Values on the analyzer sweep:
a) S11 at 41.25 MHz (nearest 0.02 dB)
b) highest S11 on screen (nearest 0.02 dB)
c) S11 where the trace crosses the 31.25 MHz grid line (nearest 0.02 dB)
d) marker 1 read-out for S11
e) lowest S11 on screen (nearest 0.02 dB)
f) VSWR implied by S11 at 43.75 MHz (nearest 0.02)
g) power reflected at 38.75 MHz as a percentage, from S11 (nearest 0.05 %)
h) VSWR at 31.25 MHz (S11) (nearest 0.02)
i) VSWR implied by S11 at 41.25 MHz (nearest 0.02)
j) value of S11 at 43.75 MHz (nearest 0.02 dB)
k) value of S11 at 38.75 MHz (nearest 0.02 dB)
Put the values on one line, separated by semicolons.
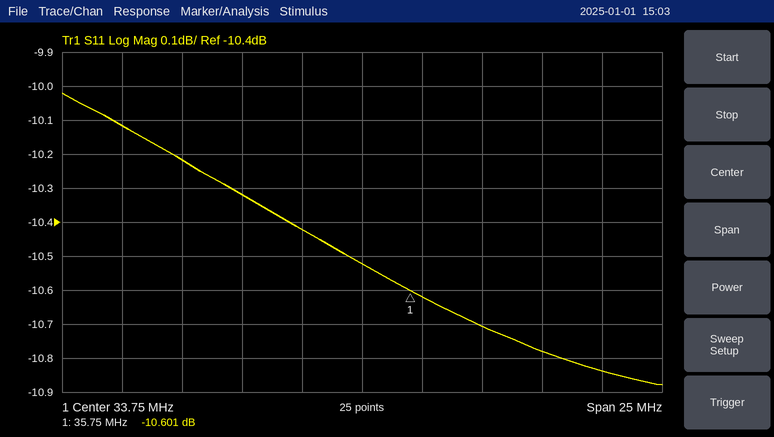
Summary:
-10.78 dB; -10.02 dB; -10.42 dB; -10.601 dB; -10.88 dB; 1.80; 8.50 %; 1.86; 1.82; -10.84 dB; -10.70 dB
